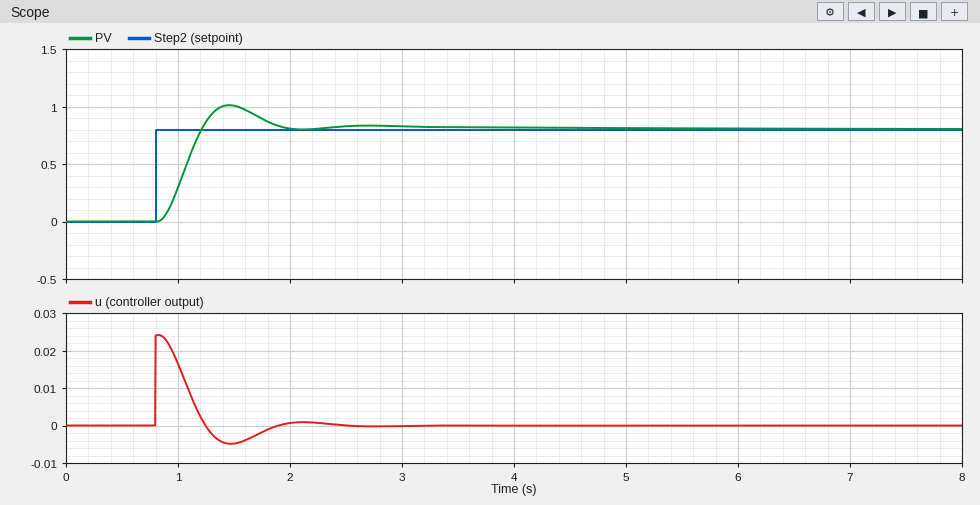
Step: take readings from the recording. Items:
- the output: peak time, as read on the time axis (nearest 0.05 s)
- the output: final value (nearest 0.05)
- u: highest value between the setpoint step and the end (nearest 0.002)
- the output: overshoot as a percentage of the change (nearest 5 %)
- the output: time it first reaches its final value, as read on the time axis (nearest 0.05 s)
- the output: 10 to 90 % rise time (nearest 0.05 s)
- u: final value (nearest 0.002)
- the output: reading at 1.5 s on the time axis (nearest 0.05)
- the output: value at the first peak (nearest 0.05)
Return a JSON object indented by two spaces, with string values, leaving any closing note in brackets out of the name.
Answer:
{
  "the output: peak time, as read on the time axis": "1.45 s",
  "the output: final value": "0.80",
  "u: highest value between the setpoint step and the end": "0.024",
  "the output: overshoot as a percentage of the change": "25 %",
  "the output: time it first reaches its final value, as read on the time axis": "1.20 s",
  "the output: 10 to 90 % rise time": "0.25 s",
  "u: final value": "0.000",
  "the output: reading at 1.5 s on the time axis": "1.00",
  "the output: value at the first peak": "1.00"
}
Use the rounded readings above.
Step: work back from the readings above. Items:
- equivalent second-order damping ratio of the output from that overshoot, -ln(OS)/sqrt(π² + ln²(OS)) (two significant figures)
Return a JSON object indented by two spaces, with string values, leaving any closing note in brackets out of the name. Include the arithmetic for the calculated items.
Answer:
{
  "equivalent second-order damping ratio of the output from that overshoot, -ln(OS)/sqrt(π² + ln²(OS))": "ln(0.25) = -1.386; 1.386 / sqrt(9.870 + 1.922) = 0.40"
}
